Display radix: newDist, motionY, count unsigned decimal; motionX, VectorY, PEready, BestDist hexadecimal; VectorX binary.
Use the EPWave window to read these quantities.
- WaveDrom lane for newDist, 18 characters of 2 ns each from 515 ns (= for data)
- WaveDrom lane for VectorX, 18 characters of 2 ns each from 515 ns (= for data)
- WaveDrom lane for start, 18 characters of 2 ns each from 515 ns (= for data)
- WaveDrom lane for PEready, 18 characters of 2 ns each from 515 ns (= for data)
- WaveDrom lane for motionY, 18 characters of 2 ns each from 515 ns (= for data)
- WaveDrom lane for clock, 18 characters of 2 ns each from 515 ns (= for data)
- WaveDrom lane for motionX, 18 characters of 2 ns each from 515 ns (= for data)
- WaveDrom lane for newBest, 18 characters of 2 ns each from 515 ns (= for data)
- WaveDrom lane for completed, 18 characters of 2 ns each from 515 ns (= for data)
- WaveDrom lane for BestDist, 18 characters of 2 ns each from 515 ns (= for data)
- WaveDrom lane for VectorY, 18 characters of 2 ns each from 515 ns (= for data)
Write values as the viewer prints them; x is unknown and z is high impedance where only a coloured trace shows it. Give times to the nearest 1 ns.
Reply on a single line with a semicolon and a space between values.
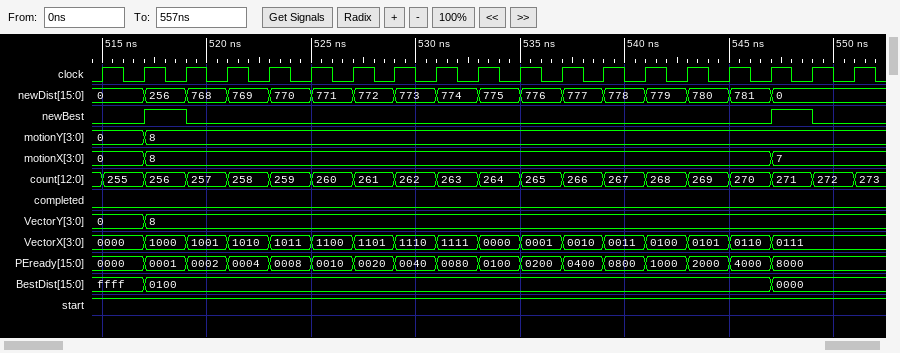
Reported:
{name: 'newDist', wave: '=================.', data: '0 256 768 769 770 771 772 773 774 775 776 777 778 779 780 781 0'}; {name: 'VectorX', wave: '=================.', data: '0000 1000 1001 1010 1011 1100 1101 1110 1111 0000 0001 0010 0011 0100 0101 0110 0111'}; {name: 'start', wave: '1.................'}; {name: 'PEready', wave: '=================.', data: '0000 0001 0002 0004 0008 0010 0020 0040 0080 0100 0200 0400 0800 1000 2000 4000 8000'}; {name: 'motionY', wave: '==................', data: '0 8'}; {name: 'clock', wave: 'p.................'}; {name: 'motionX', wave: '==..............=.', data: '0 8 7'}; {name: 'newBest', wave: '010.............10'}; {name: 'completed', wave: '0.................'}; {name: 'BestDist', wave: '==..............=.', data: 'ffff 0100 0000'}; {name: 'VectorY', wave: '==................', data: '0 8'}
